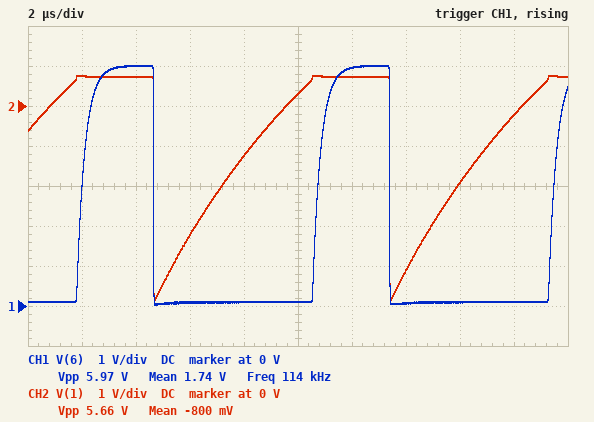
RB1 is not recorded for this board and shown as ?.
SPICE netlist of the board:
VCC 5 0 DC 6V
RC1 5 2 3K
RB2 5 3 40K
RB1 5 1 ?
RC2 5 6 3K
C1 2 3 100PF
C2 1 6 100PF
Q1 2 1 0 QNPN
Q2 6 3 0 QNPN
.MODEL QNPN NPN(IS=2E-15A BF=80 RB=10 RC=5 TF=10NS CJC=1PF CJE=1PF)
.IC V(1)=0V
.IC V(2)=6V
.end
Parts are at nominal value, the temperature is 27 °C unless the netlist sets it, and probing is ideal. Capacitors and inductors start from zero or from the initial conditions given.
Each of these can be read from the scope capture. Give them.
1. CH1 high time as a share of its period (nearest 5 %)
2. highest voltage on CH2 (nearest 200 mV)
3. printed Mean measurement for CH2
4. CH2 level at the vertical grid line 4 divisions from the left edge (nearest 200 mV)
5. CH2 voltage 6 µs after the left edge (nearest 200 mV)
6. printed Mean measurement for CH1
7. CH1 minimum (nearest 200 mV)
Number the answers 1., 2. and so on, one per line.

1. 30 %
2. 800 mV
3. -800 mV
4. -1.2 V
5. -3.2 V
6. 1.74 V
7. 0 V
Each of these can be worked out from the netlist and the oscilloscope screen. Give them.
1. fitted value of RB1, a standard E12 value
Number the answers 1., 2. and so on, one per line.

1. 82 kΩ
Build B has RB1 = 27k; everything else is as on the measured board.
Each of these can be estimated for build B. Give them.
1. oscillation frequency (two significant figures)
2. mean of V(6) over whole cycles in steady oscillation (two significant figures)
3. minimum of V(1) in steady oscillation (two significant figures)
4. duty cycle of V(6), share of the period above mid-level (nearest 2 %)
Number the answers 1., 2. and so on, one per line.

1. 210 kHz
2. 3.3 V
3. -4.8 V
4. 56 %
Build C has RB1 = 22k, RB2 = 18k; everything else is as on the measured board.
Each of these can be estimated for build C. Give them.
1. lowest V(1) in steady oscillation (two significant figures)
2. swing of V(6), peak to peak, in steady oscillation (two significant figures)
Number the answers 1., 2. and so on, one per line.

1. -4.7 V
2. 5.9 V
